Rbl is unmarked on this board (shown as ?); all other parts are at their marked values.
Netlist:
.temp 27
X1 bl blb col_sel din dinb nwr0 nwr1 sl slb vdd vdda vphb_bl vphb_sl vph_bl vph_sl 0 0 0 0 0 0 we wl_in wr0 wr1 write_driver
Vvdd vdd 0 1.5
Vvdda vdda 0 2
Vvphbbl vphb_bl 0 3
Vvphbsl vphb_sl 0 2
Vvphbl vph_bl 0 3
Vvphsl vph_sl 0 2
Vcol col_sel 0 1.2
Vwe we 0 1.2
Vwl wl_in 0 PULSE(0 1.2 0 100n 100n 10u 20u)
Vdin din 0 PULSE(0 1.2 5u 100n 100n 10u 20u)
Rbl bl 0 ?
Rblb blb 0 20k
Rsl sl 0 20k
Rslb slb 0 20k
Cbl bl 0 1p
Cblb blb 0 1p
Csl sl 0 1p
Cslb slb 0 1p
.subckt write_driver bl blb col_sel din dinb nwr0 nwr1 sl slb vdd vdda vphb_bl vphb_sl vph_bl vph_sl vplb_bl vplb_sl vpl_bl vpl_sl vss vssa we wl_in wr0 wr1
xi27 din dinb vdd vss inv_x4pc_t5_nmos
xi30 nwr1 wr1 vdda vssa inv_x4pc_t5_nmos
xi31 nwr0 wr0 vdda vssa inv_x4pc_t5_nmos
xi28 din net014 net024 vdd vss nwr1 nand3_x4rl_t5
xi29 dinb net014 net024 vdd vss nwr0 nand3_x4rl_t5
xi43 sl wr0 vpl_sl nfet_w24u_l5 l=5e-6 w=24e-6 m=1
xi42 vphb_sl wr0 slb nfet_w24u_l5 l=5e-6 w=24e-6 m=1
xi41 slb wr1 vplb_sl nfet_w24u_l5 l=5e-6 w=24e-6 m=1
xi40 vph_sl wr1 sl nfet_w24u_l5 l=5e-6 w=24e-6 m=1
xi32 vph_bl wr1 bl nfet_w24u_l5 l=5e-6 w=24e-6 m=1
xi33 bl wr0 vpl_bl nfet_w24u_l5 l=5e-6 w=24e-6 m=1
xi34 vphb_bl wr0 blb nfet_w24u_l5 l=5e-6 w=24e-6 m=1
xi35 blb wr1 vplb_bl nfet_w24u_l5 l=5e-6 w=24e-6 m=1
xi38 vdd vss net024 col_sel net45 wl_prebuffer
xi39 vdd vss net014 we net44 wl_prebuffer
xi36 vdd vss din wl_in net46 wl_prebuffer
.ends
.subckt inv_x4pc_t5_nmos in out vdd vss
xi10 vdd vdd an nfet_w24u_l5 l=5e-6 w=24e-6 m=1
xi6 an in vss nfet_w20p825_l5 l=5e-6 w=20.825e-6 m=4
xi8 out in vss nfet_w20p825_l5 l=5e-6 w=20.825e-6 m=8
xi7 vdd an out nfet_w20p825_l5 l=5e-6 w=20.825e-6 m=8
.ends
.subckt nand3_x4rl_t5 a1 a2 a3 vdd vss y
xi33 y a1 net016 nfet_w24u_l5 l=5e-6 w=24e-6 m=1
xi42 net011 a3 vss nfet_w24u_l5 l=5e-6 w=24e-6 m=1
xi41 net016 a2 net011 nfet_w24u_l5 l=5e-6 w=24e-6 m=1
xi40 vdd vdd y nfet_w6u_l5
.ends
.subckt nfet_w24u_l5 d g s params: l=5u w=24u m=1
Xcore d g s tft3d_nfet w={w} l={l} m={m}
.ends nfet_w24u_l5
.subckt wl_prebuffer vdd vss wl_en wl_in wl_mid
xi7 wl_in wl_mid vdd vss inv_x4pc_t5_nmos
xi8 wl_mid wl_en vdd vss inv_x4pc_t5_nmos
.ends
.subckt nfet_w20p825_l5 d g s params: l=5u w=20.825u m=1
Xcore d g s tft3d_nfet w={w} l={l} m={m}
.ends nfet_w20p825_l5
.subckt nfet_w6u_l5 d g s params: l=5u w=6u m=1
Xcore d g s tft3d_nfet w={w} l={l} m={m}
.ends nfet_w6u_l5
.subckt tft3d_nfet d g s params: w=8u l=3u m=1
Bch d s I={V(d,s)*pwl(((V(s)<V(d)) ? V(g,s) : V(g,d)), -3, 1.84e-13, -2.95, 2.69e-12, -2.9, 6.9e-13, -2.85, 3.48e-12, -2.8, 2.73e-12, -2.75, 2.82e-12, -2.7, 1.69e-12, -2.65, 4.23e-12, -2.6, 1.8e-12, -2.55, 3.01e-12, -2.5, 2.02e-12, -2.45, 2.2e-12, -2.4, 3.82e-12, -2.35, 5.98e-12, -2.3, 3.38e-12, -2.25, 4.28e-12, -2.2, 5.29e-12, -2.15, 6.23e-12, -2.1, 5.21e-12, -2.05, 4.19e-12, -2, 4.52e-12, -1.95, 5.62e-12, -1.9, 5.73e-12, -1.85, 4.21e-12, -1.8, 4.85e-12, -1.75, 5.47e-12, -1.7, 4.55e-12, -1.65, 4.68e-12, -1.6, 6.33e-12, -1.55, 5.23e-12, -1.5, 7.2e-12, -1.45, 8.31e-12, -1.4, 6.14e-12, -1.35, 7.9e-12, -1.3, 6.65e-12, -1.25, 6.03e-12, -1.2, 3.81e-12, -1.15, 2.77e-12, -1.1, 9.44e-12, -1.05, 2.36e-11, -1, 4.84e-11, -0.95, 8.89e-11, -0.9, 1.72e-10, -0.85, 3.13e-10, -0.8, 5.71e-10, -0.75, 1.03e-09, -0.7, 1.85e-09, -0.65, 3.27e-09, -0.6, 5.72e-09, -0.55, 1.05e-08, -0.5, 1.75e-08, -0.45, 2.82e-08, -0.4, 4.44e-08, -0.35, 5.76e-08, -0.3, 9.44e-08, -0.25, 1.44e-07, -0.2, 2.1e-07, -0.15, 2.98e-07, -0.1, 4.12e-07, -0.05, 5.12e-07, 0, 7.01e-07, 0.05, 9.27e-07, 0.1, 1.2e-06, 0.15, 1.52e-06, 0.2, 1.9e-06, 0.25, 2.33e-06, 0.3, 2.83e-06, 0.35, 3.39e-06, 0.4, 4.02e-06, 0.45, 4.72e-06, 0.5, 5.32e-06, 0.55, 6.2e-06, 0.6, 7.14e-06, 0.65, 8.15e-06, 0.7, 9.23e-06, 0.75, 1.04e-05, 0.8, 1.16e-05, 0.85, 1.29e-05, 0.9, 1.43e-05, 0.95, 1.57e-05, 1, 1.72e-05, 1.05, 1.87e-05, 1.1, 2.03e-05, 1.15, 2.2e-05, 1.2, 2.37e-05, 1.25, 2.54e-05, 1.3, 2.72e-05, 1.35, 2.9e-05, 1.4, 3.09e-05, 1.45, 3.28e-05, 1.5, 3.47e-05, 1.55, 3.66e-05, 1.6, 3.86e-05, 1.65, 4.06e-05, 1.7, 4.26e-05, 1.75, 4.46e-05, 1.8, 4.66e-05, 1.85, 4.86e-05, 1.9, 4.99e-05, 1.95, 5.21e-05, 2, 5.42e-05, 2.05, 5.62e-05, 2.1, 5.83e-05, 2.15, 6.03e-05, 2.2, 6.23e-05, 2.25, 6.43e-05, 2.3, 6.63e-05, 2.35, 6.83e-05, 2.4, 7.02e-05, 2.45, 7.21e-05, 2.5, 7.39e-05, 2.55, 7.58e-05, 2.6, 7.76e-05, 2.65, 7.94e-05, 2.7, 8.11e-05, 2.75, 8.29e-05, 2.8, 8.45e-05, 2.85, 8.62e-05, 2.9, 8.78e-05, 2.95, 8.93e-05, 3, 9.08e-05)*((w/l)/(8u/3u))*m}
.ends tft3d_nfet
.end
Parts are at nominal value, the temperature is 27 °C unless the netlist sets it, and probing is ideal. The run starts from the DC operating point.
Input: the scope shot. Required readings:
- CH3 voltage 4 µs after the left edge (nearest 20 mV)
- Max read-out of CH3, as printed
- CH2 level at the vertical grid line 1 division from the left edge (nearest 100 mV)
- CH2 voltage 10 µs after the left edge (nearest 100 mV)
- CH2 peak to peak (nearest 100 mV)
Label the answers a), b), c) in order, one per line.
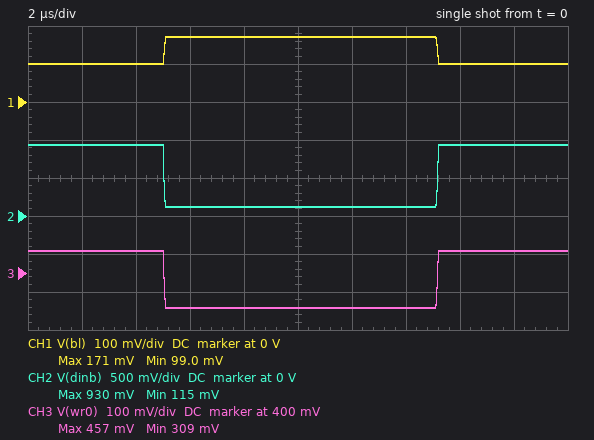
a) 460 mV
b) 457 mV
c) 900 mV
d) 100 mV
e) 800 mV
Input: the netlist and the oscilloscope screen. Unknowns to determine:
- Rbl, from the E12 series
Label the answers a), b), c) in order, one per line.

a) 12 kΩ
